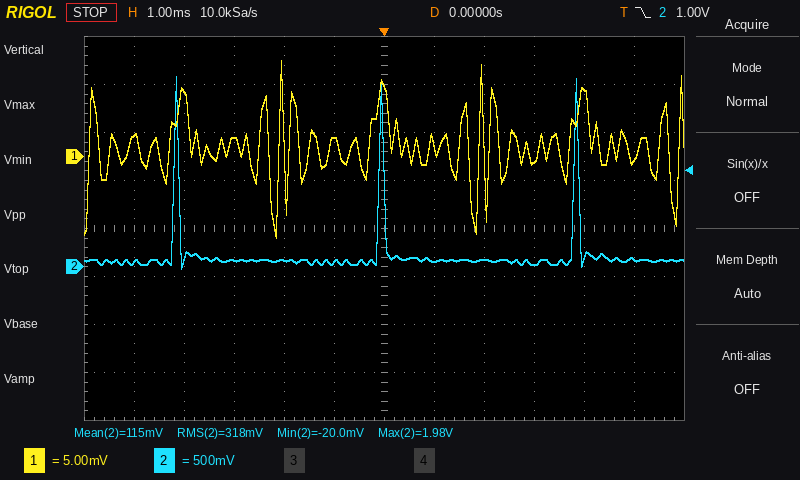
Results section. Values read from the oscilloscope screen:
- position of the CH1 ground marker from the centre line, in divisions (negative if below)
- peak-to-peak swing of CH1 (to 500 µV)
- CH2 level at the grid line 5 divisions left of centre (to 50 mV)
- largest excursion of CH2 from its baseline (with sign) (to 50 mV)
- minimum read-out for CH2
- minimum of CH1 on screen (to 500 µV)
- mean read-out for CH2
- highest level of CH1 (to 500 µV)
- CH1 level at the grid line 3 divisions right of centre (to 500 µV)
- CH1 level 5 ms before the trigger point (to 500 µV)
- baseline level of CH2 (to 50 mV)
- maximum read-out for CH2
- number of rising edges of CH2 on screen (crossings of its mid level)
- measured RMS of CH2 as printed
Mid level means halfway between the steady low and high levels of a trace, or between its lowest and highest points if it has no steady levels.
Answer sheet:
+1.5 div
18.5 mV
50 mV
+1.90 V
-20.0 mV
-8.5 mV
115 mV
10.0 mV
-500 µV
2.0 mV
50 mV
1.98 V
3
318 mV
